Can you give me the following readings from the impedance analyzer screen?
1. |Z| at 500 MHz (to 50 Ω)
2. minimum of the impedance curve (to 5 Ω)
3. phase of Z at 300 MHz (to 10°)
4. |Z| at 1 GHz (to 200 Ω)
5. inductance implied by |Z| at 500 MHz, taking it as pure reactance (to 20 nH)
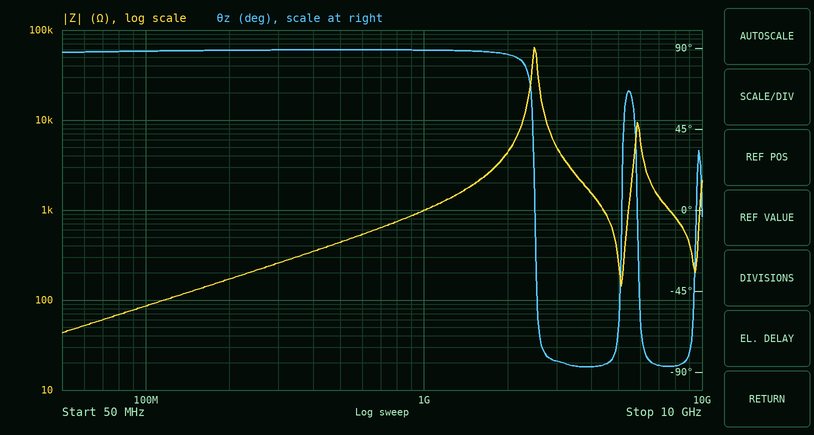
450 Ω
45 Ω
90°
1.0 kΩ
140 nH
